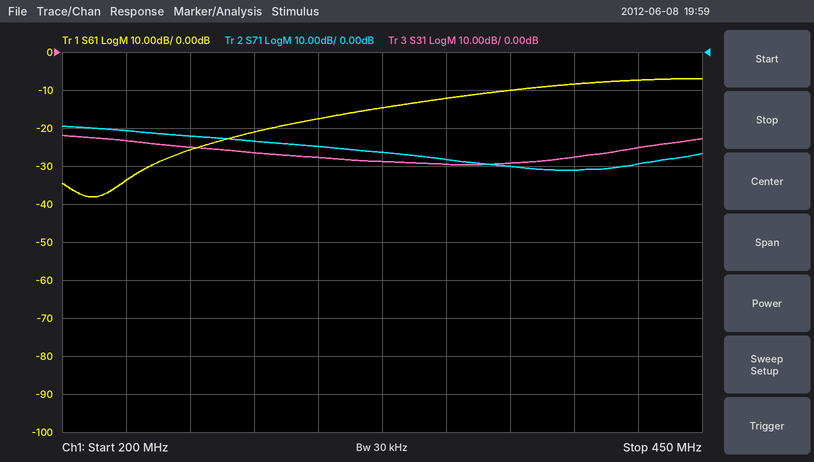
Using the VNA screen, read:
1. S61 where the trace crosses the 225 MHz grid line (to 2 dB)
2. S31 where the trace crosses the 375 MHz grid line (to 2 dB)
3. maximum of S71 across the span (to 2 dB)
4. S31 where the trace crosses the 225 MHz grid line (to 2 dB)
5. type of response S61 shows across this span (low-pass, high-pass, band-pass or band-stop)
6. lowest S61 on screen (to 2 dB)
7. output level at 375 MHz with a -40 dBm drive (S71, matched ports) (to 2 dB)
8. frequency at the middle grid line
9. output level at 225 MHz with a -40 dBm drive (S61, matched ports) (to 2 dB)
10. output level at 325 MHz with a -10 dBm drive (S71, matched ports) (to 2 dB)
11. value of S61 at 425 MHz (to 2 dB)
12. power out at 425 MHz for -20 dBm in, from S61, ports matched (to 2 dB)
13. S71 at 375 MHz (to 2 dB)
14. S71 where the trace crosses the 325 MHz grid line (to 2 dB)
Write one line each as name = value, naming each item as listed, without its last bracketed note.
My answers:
S61 where the trace crosses the 225 MHz grid line = -34 dB
S31 where the trace crosses the 375 MHz grid line = -30 dB
maximum of S71 across the span = -20 dB
S31 where the trace crosses the 225 MHz grid line = -24 dB
type of response S61 shows across this span = high-pass
lowest S61 on screen = -38 dB
output level at 375 MHz with a -40 dBm drive (S71, matched ports) = -70 dBm
frequency at the middle grid line = 325 MHz
output level at 225 MHz with a -40 dBm drive (S61, matched ports) = -74 dBm
output level at 325 MHz with a -10 dBm drive (S71, matched ports) = -36 dBm
value of S61 at 425 MHz = -8 dB
power out at 425 MHz for -20 dBm in, from S61, ports matched = -28 dBm
S71 at 375 MHz = -30 dB
S71 where the trace crosses the 325 MHz grid line = -26 dB
